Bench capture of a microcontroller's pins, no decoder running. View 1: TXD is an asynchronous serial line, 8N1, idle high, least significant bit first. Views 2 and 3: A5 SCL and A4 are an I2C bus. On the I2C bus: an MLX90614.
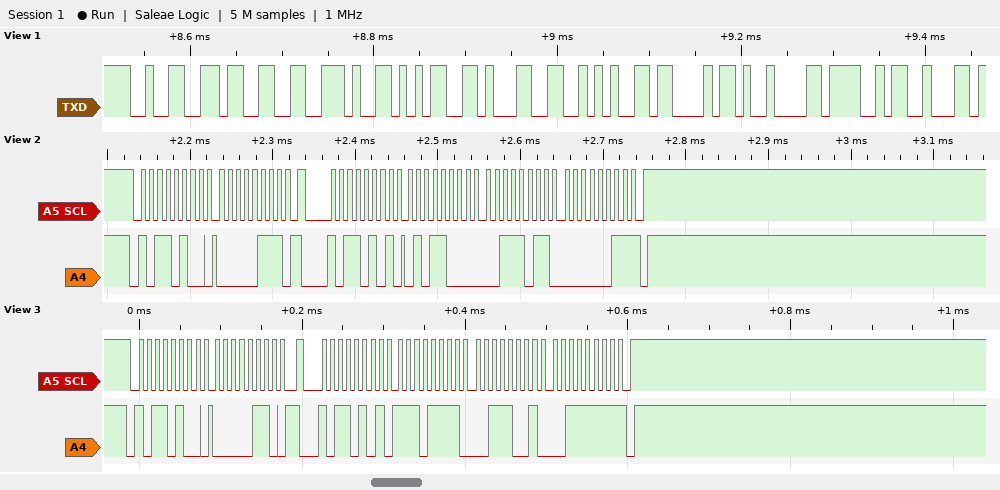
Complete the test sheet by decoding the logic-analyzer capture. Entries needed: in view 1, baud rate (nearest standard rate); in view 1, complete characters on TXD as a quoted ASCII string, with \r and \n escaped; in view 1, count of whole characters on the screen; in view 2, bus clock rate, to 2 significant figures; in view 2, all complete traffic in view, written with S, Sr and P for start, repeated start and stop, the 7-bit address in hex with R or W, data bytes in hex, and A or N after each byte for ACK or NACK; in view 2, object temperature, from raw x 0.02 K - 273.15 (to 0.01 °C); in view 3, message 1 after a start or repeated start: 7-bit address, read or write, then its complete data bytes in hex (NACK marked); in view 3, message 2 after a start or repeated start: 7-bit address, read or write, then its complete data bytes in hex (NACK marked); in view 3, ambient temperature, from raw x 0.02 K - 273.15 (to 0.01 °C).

115200 baud
"23.51*C\tOb"
10
100 kHz
S 5AW A 07 A Sr 5AR A 58 A 3B A 03 N P
30.69 °C
0x5A write: 06
0x5A read: EF 39 3F NACK
23.47 °C
